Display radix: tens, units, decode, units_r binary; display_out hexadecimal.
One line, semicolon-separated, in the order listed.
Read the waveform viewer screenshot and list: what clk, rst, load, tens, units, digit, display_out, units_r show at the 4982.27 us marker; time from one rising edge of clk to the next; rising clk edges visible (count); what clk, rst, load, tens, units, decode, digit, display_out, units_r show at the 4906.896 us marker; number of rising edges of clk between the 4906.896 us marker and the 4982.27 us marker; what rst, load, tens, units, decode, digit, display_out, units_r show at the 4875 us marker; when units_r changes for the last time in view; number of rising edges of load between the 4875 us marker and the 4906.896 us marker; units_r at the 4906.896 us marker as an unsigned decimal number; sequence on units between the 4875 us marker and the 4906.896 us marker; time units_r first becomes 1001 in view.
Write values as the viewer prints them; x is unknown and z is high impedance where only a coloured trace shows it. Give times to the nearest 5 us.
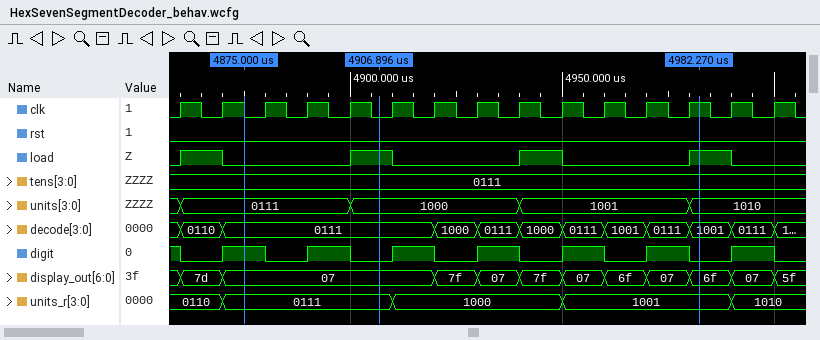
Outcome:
clk=1, rst=0, load=1, tens=0111, units=1010, digit=0, display_out=6f, units_r=1001; 10 us; 15; clk=0, rst=0, load=1, tens=0111, units=1000, decode=0111, digit=0, display_out=07, units_r=0111; 8; rst=0, load=0, tens=0111, units=0111, decode=0111, digit=1, display_out=07, units_r=0111; 4990 us; 1; 7; 0111, 1000; 4950 us
